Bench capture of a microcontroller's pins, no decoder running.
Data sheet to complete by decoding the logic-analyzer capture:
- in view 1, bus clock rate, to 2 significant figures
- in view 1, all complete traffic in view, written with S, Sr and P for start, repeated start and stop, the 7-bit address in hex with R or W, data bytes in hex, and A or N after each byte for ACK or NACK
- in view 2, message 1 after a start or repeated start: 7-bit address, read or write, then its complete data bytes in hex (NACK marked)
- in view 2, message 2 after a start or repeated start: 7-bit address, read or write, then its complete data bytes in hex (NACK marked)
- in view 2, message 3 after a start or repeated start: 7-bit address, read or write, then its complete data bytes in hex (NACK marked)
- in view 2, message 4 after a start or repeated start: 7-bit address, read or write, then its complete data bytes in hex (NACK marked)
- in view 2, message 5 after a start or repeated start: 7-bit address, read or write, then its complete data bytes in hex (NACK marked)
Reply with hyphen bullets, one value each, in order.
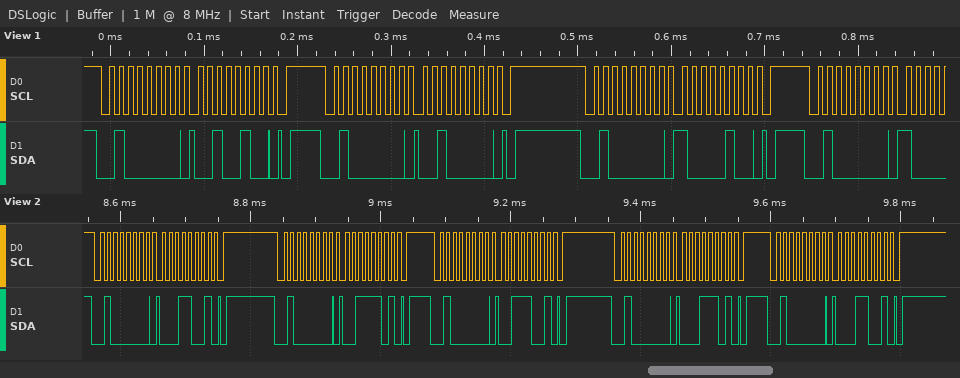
- 100 kHz
- S 20W A 24 A P S 20W A 20 A P S 20W A 84 A P S 20W A
- 0x20 write: 19
- 0x20 write: 3D
- 0x20 write: 39
- 0x20 write: 1D
- 0x20 write: 19
